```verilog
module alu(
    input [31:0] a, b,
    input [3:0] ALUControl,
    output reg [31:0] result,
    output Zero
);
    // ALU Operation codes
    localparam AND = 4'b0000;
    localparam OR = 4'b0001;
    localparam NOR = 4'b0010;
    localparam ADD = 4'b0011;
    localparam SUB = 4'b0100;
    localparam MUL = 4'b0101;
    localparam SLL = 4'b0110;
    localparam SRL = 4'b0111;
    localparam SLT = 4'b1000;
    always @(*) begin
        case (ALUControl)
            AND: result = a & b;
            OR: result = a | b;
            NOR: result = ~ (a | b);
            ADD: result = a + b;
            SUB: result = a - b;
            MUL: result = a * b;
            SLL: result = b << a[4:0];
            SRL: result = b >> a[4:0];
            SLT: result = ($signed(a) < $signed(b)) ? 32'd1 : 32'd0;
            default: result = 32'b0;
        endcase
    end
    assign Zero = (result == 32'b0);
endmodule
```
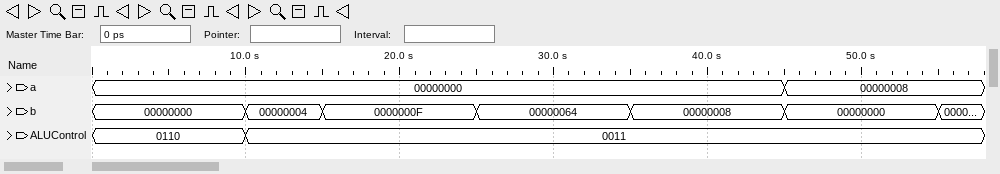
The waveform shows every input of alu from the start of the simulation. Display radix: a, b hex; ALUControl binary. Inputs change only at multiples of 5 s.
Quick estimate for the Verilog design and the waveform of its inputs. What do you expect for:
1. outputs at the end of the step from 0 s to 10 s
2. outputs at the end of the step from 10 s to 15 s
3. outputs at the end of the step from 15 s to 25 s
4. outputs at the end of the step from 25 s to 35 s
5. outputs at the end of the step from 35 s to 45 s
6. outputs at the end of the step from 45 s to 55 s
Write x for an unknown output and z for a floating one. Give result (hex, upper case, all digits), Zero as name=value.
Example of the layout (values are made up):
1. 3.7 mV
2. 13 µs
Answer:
1. result=00000000, Zero=1
2. result=00000004, Zero=0
3. result=0000000F, Zero=0
4. result=00000064, Zero=0
5. result=00000008, Zero=0
6. result=00000008, Zero=0
